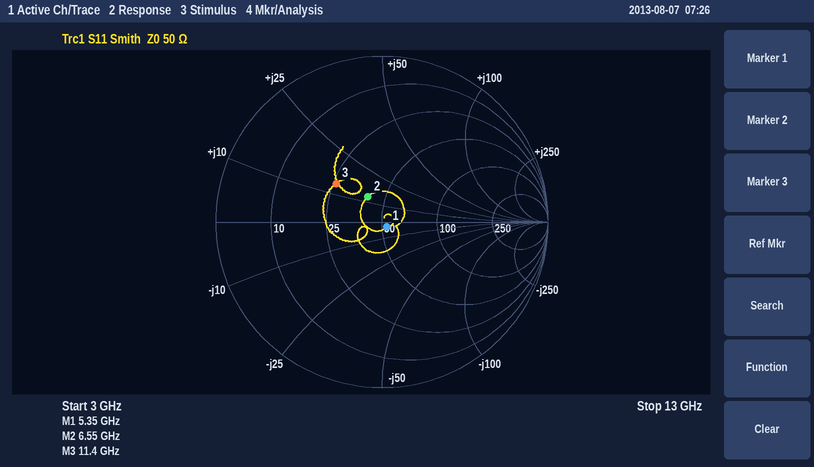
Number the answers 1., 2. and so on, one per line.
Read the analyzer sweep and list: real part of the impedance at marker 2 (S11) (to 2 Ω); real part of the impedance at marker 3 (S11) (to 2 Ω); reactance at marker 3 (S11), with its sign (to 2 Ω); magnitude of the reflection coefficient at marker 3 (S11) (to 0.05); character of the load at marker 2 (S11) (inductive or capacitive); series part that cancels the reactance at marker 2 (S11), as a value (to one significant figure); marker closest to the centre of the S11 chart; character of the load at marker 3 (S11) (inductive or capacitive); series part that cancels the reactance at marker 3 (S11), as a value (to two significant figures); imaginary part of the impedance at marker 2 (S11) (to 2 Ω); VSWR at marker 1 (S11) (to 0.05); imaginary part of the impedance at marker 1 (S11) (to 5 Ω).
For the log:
1. 40 Ω
2. 26 Ω
3. +14 Ω
4. 0.35
5. inductive
6. 2 pF
7. marker 1
8. inductive
9. 1.0 pF
10. +12 Ω
11. 1.10
12. -5 Ω
